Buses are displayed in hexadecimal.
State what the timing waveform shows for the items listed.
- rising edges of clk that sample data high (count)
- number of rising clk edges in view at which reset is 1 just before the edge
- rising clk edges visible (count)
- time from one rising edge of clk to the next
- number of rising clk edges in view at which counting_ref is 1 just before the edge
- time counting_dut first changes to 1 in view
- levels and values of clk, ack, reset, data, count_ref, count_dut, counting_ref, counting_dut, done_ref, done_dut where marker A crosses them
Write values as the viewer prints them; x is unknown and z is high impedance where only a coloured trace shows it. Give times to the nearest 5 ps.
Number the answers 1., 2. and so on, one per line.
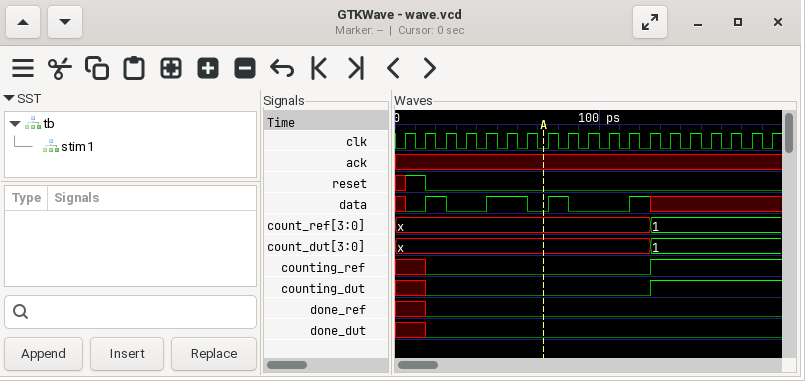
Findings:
1. 5
2. 1
3. 19
4. 10 ps
5. 6
6. 125 ps
7. clk=0, ack=x, reset=0, data=0, count_ref=x, count_dut=x, counting_ref=0, counting_dut=0, done_ref=0, done_dut=0
